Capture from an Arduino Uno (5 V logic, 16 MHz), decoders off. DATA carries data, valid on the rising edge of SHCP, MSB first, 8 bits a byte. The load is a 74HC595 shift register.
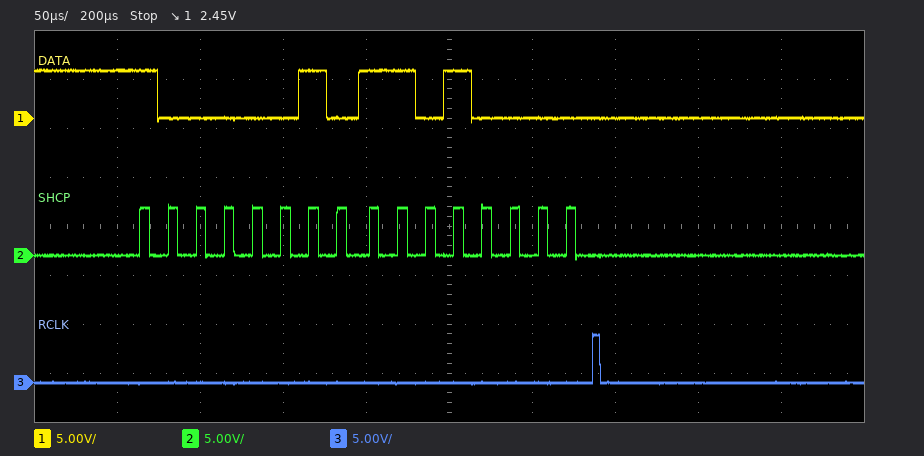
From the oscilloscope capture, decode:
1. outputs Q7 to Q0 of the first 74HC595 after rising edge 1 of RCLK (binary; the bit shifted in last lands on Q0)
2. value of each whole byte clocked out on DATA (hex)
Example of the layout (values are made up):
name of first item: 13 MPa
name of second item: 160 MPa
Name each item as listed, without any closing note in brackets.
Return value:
outputs Q7 to Q0 of the first 74HC595 after rising edge 1 of RCLK: 11010000
value of each whole byte clocked out on DATA: 0x82 0xD0
